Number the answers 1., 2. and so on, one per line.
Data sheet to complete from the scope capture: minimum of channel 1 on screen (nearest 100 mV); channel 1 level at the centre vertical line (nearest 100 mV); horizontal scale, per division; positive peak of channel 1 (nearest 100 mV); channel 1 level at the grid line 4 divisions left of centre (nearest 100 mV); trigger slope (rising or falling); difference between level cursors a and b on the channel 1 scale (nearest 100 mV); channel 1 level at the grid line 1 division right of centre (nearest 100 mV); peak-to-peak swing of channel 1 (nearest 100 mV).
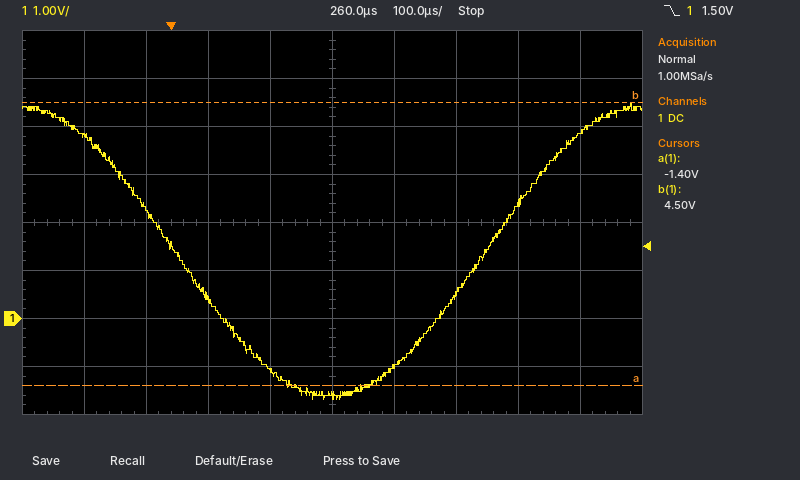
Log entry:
1. -1.7 V
2. -1.6 V
3. 100 µs
4. 4.5 V
5. 3.8 V
6. falling
7. 5.9 V
8. -1.0 V
9. 6.2 V
